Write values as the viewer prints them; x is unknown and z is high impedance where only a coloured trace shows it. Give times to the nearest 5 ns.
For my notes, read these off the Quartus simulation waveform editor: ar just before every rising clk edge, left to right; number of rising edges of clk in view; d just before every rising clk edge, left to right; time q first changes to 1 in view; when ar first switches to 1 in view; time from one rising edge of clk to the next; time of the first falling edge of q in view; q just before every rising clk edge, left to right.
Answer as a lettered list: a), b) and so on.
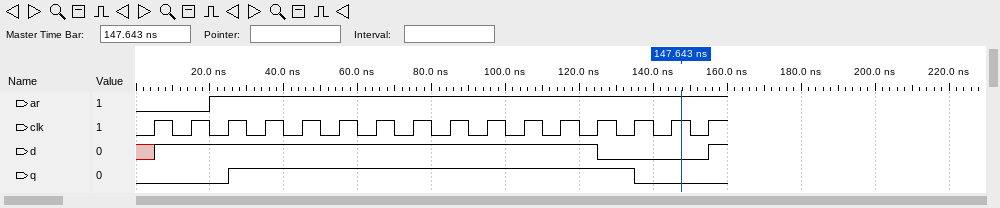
a) 0 0 1 1 1 1 1 1 1 1 1 1 1 1 1 1
b) 16
c) x 1 1 1 1 1 1 1 1 1 1 1 1 0 0 0
d) 25 ns
e) 20 ns
f) 10 ns
g) 135 ns
h) 0 0 0 1 1 1 1 1 1 1 1 1 1 1 0 0
